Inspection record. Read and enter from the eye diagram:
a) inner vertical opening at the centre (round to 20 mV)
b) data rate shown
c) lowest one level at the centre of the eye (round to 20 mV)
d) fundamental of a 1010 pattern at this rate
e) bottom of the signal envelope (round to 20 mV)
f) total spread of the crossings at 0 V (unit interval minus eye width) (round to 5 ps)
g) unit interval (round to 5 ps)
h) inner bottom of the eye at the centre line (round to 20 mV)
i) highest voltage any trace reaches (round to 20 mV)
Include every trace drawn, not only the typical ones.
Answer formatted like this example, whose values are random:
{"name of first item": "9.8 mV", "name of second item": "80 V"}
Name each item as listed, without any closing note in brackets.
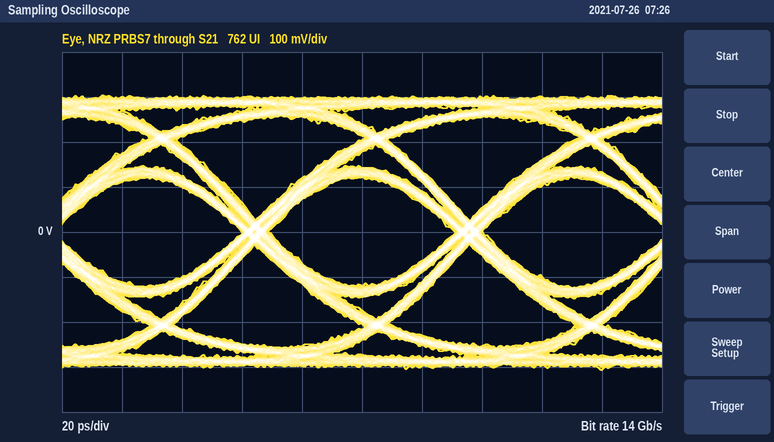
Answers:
{"inner vertical opening at the centre": "240 mV", "data rate shown": "14 Gb/s", "lowest one level at the centre of the eye": "120 mV", "fundamental of a 1010 pattern at this rate": "7 GHz", "bottom of the signal envelope": "-300 mV", "total spread of the crossings at 0 V (unit interval minus eye width)": "10 ps", "unit interval": "70 ps", "inner bottom of the eye at the centre line": "-120 mV", "highest voltage any trace reaches": "300 mV"}
